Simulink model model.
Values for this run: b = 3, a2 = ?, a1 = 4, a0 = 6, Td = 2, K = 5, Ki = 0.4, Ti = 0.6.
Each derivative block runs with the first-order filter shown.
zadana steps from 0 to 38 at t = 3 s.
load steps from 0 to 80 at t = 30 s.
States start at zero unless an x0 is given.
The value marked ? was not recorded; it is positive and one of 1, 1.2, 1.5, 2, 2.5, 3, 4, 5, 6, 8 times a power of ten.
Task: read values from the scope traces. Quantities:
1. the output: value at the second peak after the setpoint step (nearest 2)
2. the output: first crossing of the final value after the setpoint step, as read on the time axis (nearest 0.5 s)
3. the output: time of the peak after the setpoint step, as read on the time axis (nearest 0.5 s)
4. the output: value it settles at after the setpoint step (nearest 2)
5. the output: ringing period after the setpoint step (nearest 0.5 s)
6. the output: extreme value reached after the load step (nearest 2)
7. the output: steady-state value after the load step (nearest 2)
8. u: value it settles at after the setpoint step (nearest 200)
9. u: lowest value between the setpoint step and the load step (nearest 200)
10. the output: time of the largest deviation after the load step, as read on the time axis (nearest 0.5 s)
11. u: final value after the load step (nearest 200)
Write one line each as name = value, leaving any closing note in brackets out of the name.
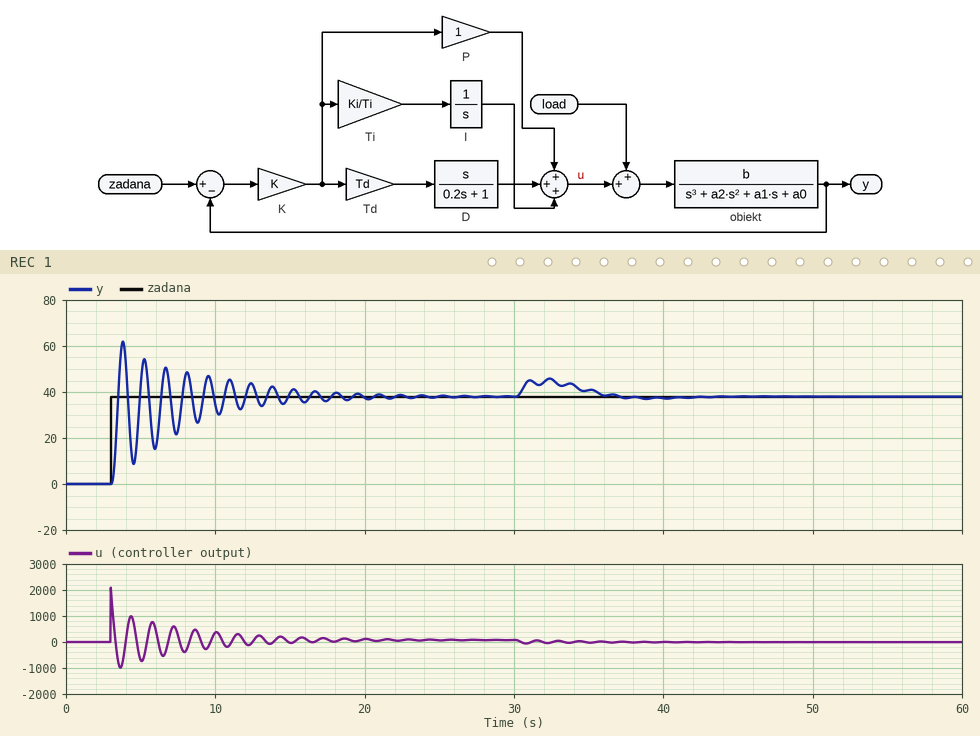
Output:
the output: value at the second peak after the setpoint step = 54
the output: first crossing of the final value after the setpoint step, as read on the time axis = 3.5 s
the output: time of the peak after the setpoint step, as read on the time axis = 4.0 s
the output: value it settles at after the setpoint step = 38
the output: ringing period after the setpoint step = 1.5 s
the output: extreme value reached after the load step = 46
the output: steady-state value after the load step = 38
u: value it settles at after the setpoint step = 0
u: lowest value between the setpoint step and the load step = -1000
the output: time of the largest deviation after the load step, as read on the time axis = 32.5 s
u: final value after the load step = 0
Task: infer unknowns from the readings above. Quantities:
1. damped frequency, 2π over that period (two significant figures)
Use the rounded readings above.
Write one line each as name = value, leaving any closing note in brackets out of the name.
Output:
damped frequency, 2π over that period = 4.2 rad/s
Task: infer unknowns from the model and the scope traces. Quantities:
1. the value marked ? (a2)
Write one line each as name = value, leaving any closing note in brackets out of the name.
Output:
the value marked ? = 5
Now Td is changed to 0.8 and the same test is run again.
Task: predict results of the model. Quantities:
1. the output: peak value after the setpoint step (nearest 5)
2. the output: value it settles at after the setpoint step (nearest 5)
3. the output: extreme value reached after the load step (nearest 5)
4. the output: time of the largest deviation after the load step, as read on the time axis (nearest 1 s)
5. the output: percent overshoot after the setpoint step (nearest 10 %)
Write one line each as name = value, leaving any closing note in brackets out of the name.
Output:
the output: peak value after the setpoint step = 55
the output: value it settles at after the setpoint step = 40
the output: extreme value reached after the load step = 50
the output: time of the largest deviation after the load step, as read on the time axis = 31 s
the output: percent overshoot after the setpoint step = 50 %
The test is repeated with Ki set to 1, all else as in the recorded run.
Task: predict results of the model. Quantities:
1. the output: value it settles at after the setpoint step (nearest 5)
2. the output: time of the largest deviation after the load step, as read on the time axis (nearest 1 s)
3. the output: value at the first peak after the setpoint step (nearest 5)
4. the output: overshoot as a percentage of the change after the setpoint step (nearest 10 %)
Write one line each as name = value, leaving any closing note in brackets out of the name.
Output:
the output: value it settles at after the setpoint step = 40
the output: time of the largest deviation after the load step, as read on the time axis = 31 s
the output: value at the first peak after the setpoint step = 65
the output: overshoot as a percentage of the change after the setpoint step = 70 %
